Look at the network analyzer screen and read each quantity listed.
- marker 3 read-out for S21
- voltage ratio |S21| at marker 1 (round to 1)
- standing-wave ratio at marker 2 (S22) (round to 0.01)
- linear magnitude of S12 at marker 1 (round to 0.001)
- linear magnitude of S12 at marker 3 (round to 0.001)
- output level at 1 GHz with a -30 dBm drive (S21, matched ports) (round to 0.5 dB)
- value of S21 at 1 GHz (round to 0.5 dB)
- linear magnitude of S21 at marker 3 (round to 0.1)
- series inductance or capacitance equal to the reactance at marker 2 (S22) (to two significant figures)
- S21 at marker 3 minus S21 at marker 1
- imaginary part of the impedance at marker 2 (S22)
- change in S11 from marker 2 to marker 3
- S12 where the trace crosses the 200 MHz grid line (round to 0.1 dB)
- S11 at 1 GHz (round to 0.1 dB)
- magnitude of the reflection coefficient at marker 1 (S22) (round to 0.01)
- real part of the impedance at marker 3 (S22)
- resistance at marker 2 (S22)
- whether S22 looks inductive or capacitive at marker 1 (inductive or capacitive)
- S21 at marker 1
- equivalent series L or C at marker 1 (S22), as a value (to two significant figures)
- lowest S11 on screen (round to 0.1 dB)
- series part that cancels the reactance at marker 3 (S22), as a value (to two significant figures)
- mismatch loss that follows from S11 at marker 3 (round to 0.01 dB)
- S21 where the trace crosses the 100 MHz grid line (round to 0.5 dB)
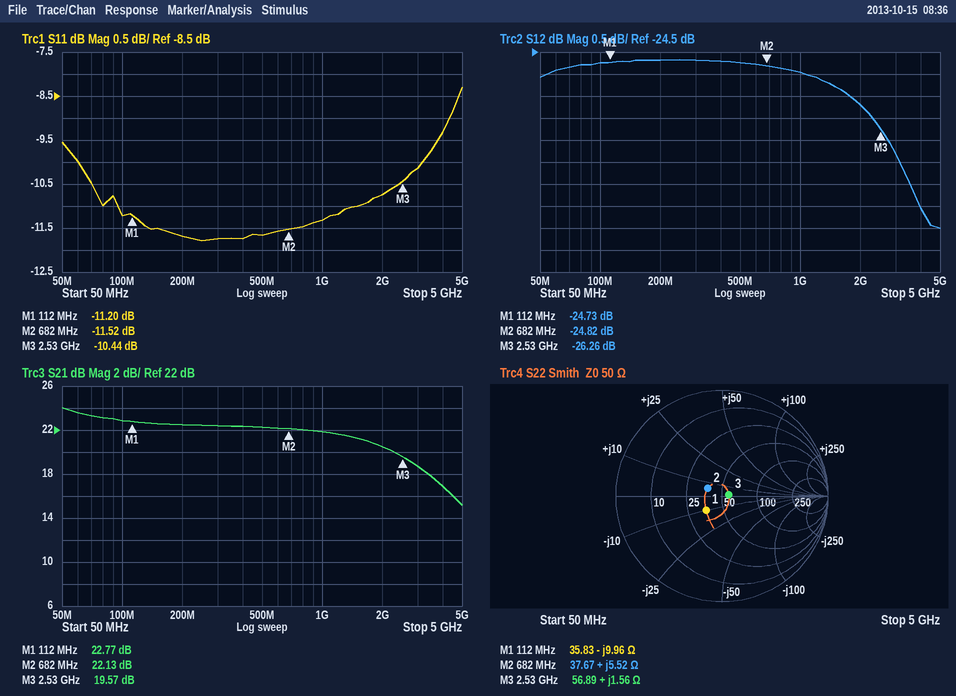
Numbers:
19.57 dB
14
1.36
0.058
0.049
-8.0 dBm
22.0 dB
9.5
1.3 nH
-3.20 dB
+5.52 Ω
1.08 dB
-24.7 dB
-11.3 dB
0.20
56.89 Ω
37.67 Ω
capacitive
22.77 dB
140 pF
-11.8 dB
40 pF
0.41 dB
23.0 dB
